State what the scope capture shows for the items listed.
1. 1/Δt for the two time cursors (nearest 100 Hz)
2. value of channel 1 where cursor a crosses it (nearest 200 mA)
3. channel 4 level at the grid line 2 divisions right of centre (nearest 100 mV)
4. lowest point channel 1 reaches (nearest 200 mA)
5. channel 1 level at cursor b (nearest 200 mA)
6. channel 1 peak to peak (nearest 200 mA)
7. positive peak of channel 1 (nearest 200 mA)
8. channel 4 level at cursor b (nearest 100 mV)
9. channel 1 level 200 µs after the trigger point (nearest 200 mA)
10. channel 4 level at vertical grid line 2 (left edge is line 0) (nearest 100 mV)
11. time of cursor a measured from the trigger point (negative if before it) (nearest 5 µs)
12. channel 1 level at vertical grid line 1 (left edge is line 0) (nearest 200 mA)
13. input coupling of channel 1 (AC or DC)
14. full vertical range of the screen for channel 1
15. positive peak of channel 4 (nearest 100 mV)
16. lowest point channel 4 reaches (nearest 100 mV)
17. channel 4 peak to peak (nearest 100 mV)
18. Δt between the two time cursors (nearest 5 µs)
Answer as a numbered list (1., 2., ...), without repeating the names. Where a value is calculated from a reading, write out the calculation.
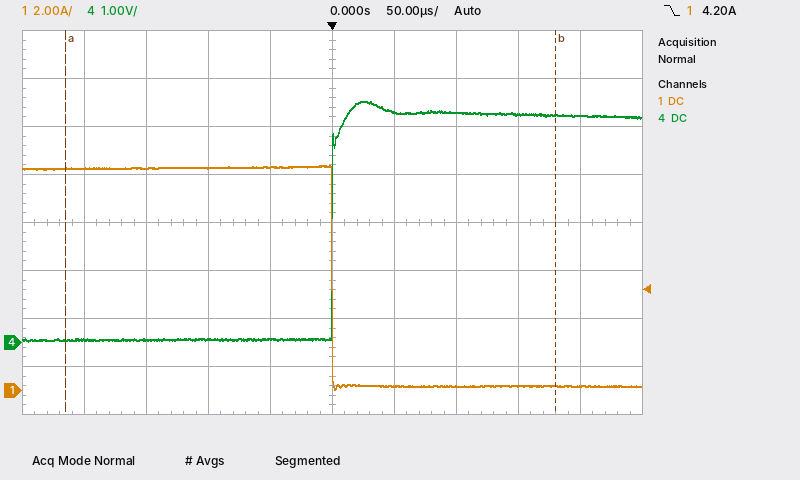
1. 1 / 395 µs ≈ 2.5 kHz
2. 9.2 A
3. 4.8 V
4. 0.0 A
5. 200 mA
6. 9.4 A − (0.0 A) = 9.4 A
7. 9.4 A
8. 4.7 V
9. 200 mA
10. 100 mV
11. -215 µs
12. 9.2 A
13. DC
14. 16 A
15. 5.0 V
16. 0.0 V
17. 5.0 V − (0.0 V) = 5.0 V
18. 395 µs
